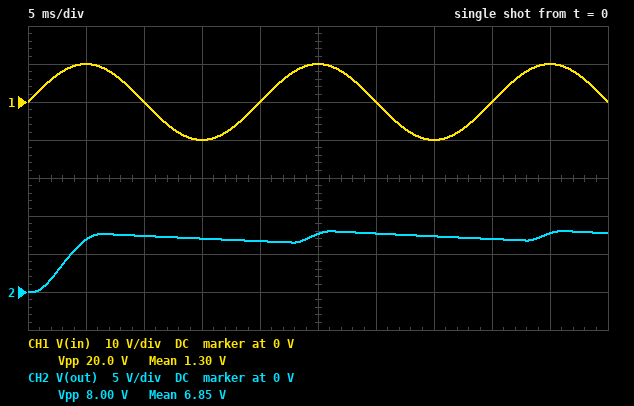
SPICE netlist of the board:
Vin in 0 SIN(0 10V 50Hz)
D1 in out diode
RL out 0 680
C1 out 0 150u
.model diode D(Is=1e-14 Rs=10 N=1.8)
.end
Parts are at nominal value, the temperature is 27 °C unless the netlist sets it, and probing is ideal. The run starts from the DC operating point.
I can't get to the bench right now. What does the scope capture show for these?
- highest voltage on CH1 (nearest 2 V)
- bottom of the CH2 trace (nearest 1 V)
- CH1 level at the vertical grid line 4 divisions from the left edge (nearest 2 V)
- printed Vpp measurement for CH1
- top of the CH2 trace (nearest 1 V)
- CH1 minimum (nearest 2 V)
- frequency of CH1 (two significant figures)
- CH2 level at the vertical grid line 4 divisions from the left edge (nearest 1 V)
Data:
10 V
0 V
0 V
20.0 V
8 V
-10 V
50 Hz
7 V
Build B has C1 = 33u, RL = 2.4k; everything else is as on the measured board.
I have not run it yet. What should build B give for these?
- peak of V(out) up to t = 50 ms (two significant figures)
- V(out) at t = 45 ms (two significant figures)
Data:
8.6 V
8.5 V
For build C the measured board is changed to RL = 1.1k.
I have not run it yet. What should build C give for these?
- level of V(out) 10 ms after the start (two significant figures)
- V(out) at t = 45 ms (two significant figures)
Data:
7.5 V
7.9 V
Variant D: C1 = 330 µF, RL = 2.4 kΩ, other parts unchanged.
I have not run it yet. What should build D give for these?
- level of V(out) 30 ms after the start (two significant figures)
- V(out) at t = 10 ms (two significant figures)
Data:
7.4 V
6.2 V
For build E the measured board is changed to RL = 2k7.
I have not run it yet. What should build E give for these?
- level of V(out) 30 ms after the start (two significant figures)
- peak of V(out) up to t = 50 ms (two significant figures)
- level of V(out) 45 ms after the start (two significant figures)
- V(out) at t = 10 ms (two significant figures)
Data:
8.1 V
8.3 V
8.2 V
7.6 V
